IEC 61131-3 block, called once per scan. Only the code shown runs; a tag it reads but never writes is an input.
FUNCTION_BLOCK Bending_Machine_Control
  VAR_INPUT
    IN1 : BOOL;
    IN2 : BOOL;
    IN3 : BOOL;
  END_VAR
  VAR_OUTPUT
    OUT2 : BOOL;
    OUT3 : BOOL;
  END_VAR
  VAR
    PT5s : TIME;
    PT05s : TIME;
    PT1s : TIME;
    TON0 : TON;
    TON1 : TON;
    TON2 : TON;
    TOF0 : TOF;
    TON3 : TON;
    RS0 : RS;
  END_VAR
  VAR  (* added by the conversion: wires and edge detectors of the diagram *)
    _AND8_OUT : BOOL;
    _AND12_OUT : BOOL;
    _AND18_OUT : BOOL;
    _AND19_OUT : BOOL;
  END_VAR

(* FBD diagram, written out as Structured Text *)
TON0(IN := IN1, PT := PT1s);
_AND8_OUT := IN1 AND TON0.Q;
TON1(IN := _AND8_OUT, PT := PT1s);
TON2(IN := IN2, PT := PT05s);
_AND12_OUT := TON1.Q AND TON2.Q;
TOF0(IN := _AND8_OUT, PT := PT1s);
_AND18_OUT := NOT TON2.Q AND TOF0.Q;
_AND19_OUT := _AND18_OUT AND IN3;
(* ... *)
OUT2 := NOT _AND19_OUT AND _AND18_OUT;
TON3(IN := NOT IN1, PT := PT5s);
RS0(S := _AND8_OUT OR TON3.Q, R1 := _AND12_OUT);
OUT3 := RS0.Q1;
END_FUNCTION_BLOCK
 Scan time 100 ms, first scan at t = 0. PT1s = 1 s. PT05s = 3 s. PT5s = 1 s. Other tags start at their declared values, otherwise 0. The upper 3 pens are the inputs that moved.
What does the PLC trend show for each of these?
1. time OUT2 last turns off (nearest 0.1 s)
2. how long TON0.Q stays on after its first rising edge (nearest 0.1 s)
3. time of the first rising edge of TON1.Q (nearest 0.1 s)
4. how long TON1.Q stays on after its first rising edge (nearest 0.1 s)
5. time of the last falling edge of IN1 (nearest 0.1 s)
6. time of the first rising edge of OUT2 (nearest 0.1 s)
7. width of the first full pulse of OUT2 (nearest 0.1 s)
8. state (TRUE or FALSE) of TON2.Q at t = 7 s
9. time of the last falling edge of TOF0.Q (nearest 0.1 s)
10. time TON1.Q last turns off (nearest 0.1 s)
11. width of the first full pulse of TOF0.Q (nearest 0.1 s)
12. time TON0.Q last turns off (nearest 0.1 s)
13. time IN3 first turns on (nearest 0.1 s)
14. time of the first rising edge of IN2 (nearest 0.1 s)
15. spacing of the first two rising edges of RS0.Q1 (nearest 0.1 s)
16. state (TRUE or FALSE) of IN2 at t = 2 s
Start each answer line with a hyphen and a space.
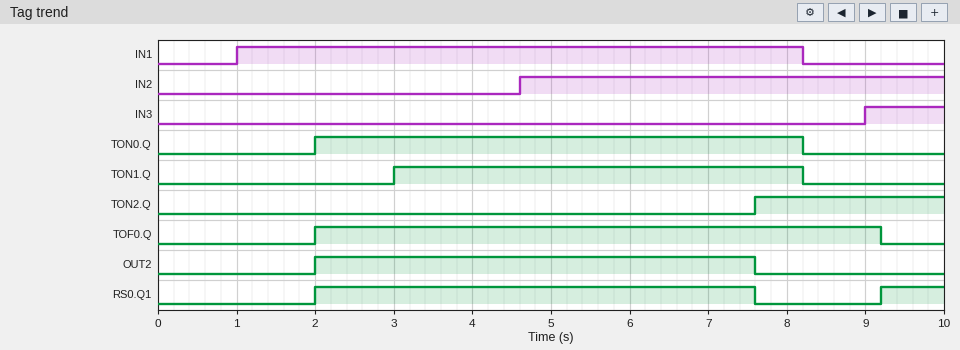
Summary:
- 7.6 s
- 6.2 s
- 3.0 s
- 5.2 s
- 8.2 s
- 2.0 s
- 5.6 s
- FALSE
- 9.2 s
- 8.2 s
- 7.2 s
- 8.2 s
- 9.0 s
- 4.6 s
- 7.2 s
- FALSE
